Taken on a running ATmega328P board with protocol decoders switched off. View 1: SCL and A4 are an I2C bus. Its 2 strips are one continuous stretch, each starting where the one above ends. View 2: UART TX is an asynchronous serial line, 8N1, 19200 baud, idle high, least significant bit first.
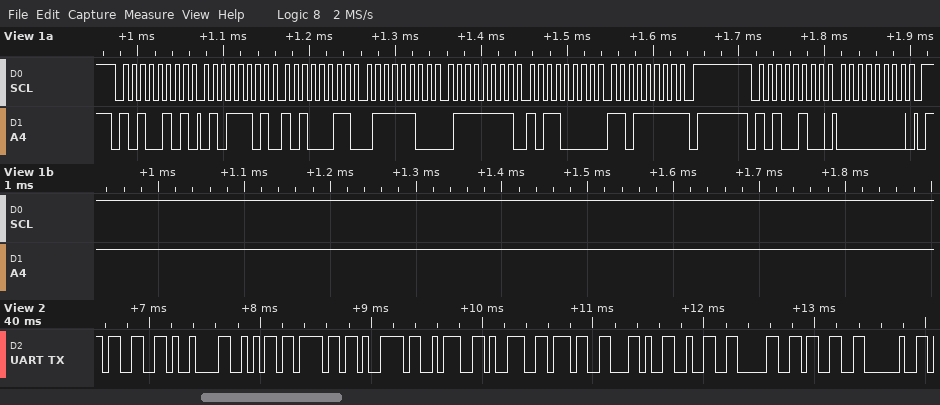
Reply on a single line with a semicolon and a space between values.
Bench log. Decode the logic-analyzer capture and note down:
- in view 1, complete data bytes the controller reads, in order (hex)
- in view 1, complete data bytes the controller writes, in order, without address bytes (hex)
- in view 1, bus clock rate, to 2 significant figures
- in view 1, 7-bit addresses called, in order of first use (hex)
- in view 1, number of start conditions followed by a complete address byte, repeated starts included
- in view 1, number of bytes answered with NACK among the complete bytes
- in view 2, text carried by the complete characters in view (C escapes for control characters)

5D A3 7C 7F B0 DF; 00; 100 kHz; 0x52; 2; 1; "3\tjoy:97,203 "
